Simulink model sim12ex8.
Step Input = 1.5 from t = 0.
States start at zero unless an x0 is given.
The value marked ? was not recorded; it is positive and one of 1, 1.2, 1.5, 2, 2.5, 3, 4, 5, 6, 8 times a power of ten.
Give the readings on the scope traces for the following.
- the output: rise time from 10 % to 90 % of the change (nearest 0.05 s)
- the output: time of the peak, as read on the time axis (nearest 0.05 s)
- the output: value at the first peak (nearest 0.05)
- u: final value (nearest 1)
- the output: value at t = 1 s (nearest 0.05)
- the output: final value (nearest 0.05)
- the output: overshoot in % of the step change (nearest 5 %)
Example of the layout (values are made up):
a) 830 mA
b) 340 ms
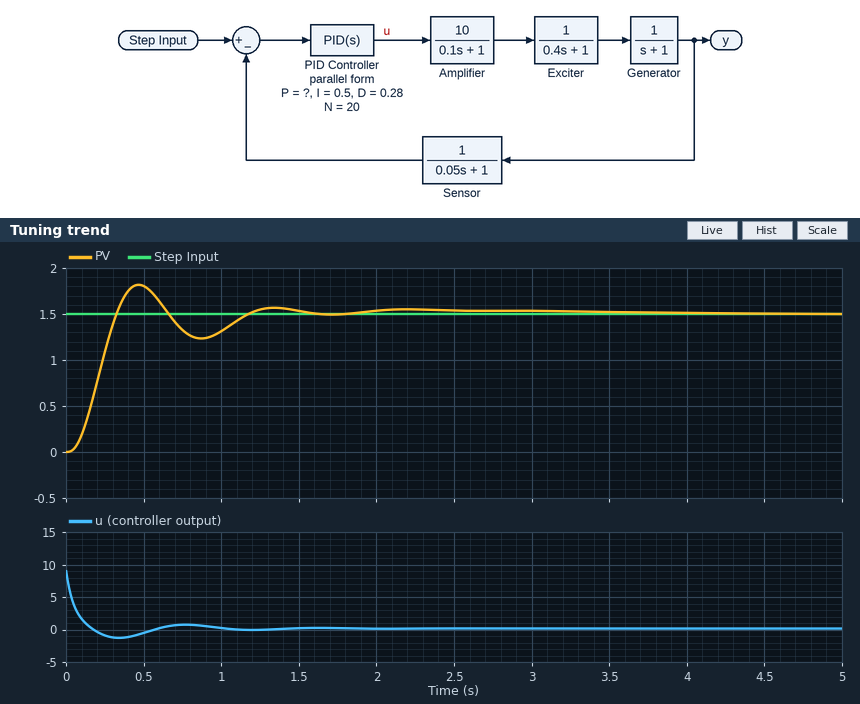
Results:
a) 0.20 s
b) 0.45 s
c) 1.80
d) 0
e) 1.30
f) 1.50
g) 20 %
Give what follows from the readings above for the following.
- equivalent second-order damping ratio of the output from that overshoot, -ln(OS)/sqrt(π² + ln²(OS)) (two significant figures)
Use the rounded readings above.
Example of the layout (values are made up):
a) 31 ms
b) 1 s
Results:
a) 0.46
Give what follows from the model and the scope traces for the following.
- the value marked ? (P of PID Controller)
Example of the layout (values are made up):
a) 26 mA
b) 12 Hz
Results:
a) 0.5
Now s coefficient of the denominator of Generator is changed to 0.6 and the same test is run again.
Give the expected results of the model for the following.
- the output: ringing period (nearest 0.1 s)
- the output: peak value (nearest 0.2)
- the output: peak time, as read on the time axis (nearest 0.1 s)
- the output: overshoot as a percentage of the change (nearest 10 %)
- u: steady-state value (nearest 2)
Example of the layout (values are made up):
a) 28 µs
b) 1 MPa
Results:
a) 0.7 s
b) 2.2
c) 0.4 s
d) 40 %
e) 0
